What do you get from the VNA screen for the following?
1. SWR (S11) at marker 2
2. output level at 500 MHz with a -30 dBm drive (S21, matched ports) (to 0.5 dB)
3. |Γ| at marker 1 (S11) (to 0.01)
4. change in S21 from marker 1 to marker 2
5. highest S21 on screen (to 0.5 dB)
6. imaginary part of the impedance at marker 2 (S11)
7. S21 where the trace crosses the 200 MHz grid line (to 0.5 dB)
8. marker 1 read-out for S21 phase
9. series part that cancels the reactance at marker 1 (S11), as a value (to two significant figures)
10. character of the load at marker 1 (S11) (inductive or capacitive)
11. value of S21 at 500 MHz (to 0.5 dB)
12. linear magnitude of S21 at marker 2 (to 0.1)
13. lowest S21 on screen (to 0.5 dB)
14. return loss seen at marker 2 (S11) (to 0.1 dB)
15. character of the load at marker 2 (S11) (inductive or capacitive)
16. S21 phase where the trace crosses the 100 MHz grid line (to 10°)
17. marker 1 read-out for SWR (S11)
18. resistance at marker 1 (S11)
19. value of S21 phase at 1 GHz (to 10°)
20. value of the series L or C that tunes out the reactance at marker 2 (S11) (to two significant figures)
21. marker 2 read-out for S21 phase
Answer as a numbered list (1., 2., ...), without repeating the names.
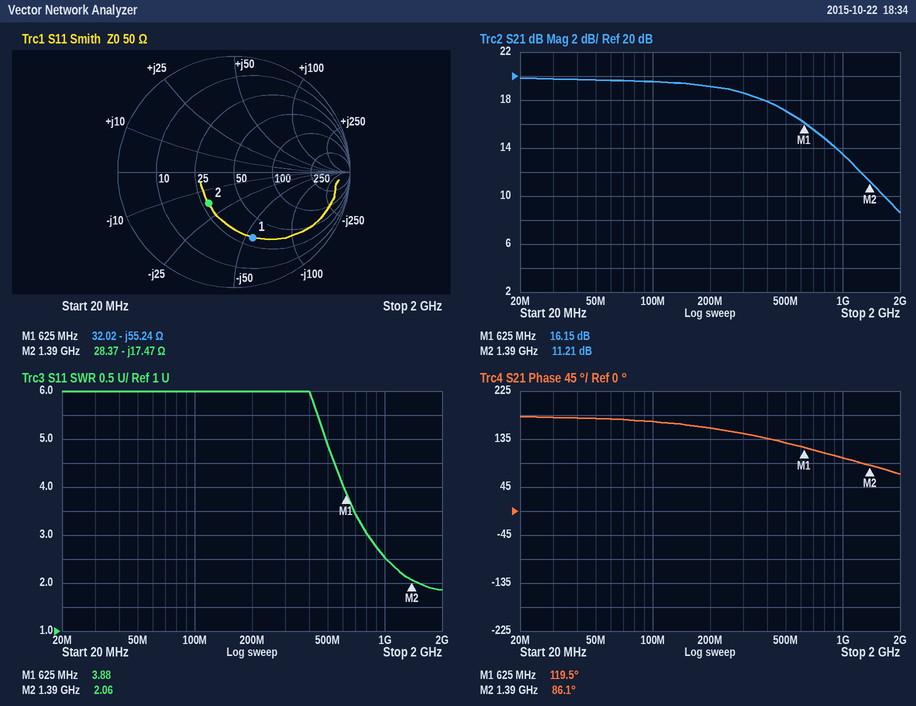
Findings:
1. 2.06
2. -13.0 dBm
3. 0.59
4. -4.94 dB
5. 20.0 dB
6. -17.47 Ω
7. 19.0 dB
8. 119.5°
9. 14 nH
10. capacitive
11. 17.0 dB
12. 3.6
13. 8.5 dB
14. 9.2 dB
15. capacitive
16. 170°
17. 3.88
18. 32.02 Ω
19. 100°
20. 2.0 nH
21. 86.1°
